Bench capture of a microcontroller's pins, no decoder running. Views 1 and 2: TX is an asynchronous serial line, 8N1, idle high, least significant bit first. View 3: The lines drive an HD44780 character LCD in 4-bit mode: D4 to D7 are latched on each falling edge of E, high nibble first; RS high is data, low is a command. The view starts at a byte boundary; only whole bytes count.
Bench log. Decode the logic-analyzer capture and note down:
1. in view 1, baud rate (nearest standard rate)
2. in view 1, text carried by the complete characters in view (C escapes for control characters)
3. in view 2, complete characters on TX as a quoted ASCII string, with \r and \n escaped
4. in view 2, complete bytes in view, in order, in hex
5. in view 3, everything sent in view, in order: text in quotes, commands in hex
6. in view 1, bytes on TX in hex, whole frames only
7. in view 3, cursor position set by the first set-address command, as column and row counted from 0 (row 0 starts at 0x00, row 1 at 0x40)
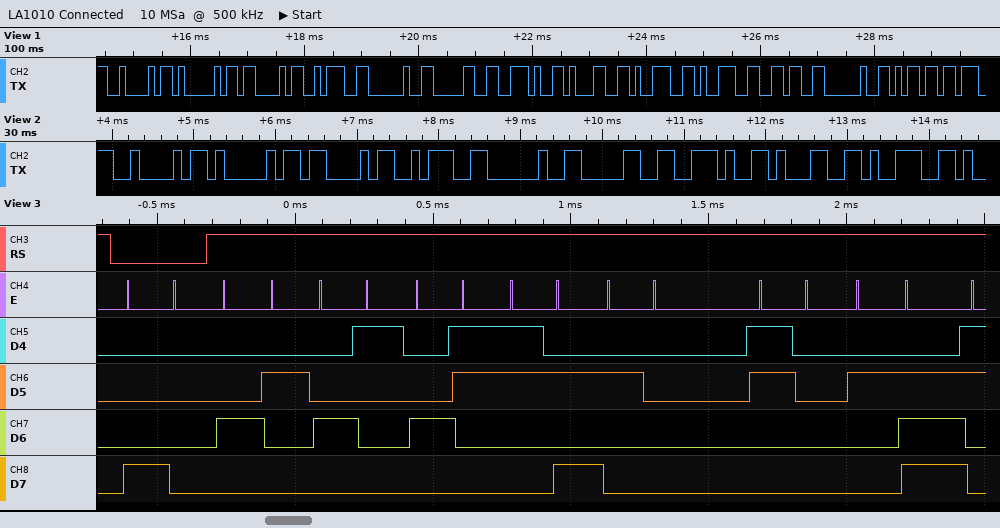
9600 baud
"BAC: 0.1996 m"
"BAC: 0.19"
42 41 43 3A 20 30 2E 31 39
0x80 "BAC: 0."
42 41 43 3A 20 30 2E 31 39 39 36 20 6D
column 0, row 0
